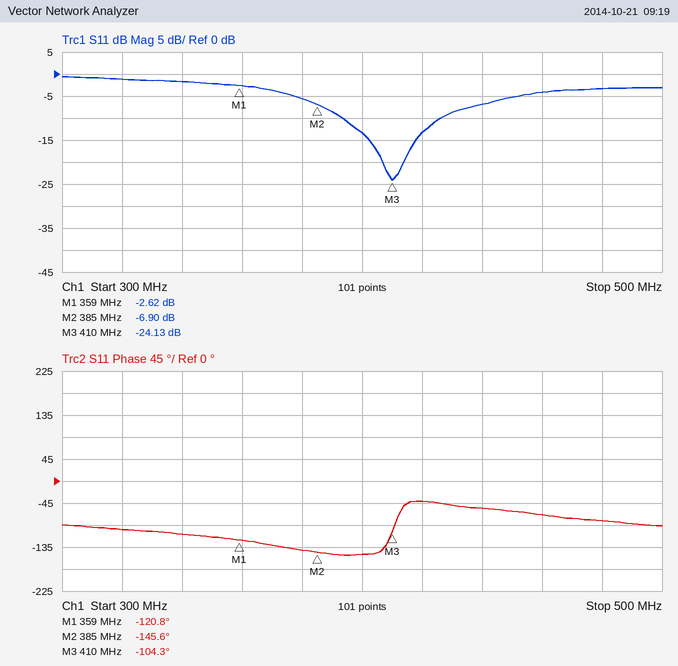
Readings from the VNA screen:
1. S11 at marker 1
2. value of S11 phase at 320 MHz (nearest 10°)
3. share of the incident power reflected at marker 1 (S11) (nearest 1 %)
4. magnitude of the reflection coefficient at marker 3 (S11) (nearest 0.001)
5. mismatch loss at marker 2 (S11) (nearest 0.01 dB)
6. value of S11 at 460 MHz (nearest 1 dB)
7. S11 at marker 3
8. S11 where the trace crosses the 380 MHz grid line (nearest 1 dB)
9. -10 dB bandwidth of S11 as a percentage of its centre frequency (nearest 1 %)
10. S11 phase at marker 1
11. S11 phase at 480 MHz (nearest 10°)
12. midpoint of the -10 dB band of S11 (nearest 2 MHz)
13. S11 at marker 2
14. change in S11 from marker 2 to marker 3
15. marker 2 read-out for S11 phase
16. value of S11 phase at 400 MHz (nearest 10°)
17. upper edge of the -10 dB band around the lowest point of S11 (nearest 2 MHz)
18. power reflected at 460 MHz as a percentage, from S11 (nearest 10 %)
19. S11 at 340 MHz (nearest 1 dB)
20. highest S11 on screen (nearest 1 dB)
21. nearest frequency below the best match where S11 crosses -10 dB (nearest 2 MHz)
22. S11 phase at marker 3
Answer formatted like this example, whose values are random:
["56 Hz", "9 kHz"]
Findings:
["-2.62 dB", "-100°", "55 %", "0.062", "0.99 dB", "-4 dB", "-24.13 dB", "-6 dB", "8 %", "-120.8°", "-80°", "410 MHz", "-6.90 dB", "-17.23 dB", "-145.6°", "-150°", "426 MHz", "40 %", "-2 dB", "-1 dB", "394 MHz", "-104.3°"]
